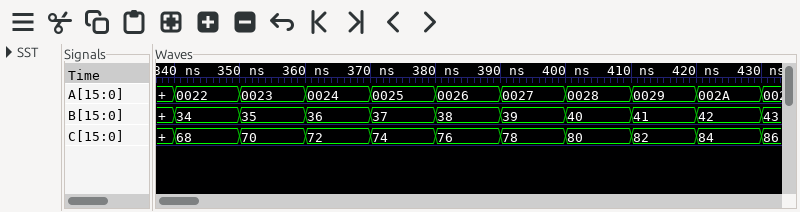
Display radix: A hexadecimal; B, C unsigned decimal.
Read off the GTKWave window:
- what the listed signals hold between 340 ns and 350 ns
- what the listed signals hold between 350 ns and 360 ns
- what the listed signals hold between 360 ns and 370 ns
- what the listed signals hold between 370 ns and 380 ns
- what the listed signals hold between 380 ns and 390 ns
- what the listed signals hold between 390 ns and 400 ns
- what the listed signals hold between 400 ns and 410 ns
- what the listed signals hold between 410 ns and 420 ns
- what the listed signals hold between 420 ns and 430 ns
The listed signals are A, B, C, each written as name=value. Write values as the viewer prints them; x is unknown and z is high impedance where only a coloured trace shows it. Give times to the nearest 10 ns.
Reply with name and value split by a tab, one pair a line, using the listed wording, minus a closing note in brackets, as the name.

what the listed signals hold between 340 ns and 350 ns	A=0022, B=34, C=68
what the listed signals hold between 350 ns and 360 ns	A=0023, B=35, C=70
what the listed signals hold between 360 ns and 370 ns	A=0024, B=36, C=72
what the listed signals hold between 370 ns and 380 ns	A=0025, B=37, C=74
what the listed signals hold between 380 ns and 390 ns	A=0026, B=38, C=76
what the listed signals hold between 390 ns and 400 ns	A=0027, B=39, C=78
what the listed signals hold between 400 ns and 410 ns	A=0028, B=40, C=80
what the listed signals hold between 410 ns and 420 ns	A=0029, B=41, C=82
what the listed signals hold between 420 ns and 430 ns	A=002A, B=42, C=84
